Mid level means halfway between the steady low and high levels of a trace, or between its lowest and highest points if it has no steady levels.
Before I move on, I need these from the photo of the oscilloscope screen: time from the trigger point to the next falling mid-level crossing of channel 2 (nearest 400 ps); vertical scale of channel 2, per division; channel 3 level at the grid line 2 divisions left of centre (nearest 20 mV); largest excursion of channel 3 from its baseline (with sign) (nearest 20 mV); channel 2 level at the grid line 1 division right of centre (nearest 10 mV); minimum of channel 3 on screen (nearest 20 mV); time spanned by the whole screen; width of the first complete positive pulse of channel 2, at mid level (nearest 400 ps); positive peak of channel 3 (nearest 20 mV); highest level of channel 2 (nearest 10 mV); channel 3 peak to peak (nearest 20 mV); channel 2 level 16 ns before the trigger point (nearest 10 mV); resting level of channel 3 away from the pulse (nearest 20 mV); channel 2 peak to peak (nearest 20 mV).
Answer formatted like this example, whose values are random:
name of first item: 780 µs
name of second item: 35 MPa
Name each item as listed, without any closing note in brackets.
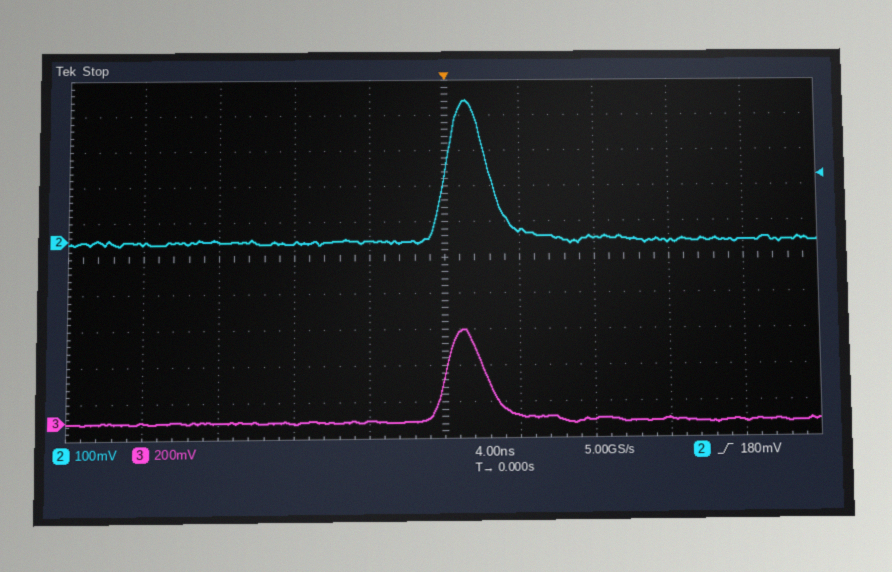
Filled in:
time from the trigger point to the next falling mid-level crossing of channel 2: 2.4 ns
vertical scale of channel 2, per division: 100 mV
channel 3 level at the grid line 2 divisions left of centre: -20 mV
largest excursion of channel 3 from its baseline (with sign): +500 mV
channel 2 level at the grid line 1 division right of centre: 30 mV
minimum of channel 3 on screen: -20 mV
time spanned by the whole screen: 40 ns
width of the first complete positive pulse of channel 2, at mid level: 2.4 ns
positive peak of channel 3: 500 mV
highest level of channel 2: 390 mV
channel 3 peak to peak: 520 mV
channel 2 level 16 ns before the trigger point: -10 mV
resting level of channel 3 away from the pulse: 0 mV
channel 2 peak to peak: 400 mV
